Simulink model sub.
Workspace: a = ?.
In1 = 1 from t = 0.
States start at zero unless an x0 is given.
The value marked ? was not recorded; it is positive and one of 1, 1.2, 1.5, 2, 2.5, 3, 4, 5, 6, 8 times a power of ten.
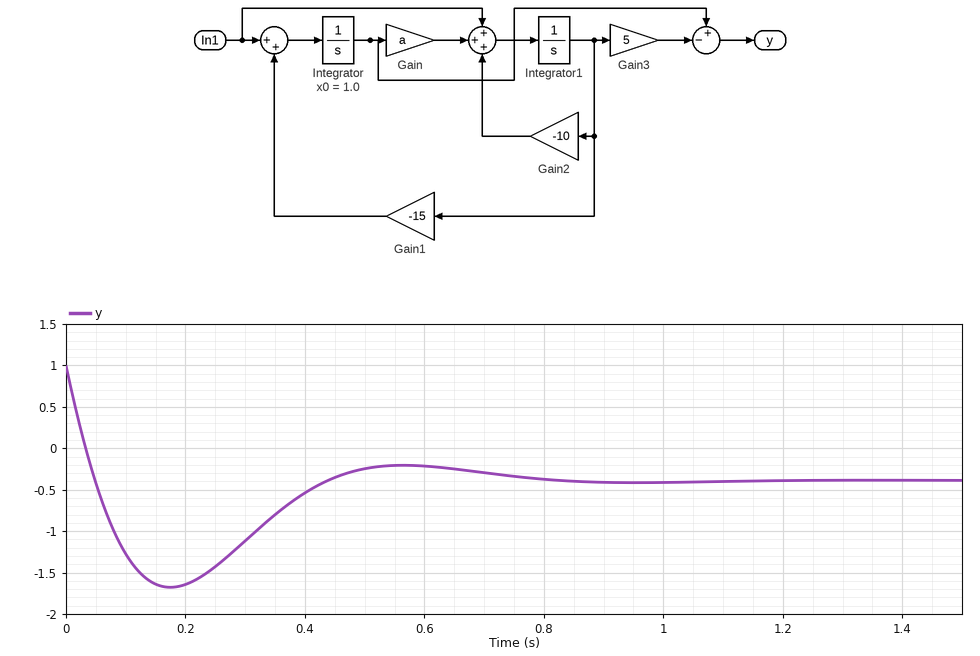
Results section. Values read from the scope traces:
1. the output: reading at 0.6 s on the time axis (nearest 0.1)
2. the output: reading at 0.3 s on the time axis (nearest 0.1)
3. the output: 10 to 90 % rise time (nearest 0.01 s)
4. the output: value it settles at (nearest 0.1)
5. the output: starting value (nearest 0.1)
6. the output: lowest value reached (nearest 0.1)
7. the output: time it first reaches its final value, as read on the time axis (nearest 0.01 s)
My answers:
-0.2
-1.1
0.04 s
-0.4
1.0
-1.7
0.05 s
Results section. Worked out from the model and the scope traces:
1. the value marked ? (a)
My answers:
6
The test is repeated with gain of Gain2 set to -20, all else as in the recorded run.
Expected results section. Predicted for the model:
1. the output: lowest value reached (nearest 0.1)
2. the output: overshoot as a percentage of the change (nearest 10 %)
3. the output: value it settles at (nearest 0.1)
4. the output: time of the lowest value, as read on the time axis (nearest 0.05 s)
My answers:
-0.7
30 %
-0.3
0.15 s
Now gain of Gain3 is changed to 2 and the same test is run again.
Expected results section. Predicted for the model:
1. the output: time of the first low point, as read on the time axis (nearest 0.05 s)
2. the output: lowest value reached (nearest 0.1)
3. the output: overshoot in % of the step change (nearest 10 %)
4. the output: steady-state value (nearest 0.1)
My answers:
0.25 s
-0.6
30 %
-0.2
